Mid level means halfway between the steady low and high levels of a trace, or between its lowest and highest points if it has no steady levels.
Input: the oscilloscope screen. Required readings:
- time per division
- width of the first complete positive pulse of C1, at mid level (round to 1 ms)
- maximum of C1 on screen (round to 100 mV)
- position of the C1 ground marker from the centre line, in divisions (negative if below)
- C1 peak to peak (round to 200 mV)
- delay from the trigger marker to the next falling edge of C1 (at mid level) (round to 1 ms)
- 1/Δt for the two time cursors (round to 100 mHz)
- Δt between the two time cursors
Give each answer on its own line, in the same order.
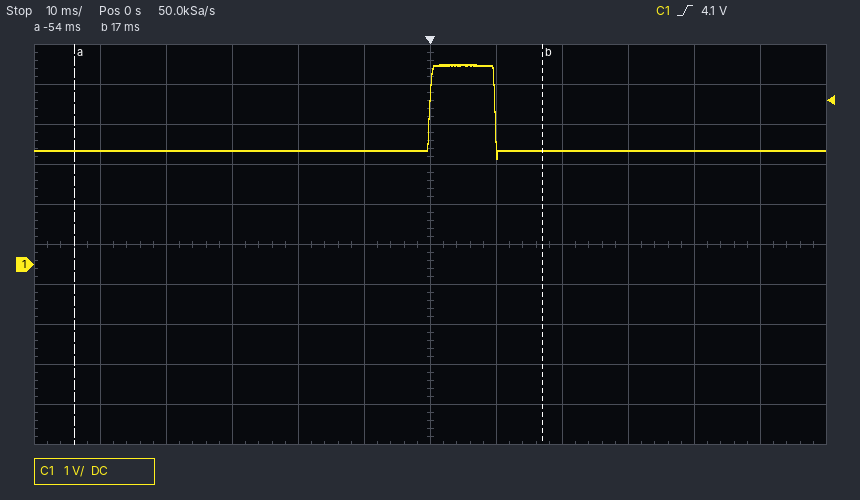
10 ms
10 ms
5.0 V
-0.5 div
2.4 V
10 ms
14.1 Hz
71 ms
